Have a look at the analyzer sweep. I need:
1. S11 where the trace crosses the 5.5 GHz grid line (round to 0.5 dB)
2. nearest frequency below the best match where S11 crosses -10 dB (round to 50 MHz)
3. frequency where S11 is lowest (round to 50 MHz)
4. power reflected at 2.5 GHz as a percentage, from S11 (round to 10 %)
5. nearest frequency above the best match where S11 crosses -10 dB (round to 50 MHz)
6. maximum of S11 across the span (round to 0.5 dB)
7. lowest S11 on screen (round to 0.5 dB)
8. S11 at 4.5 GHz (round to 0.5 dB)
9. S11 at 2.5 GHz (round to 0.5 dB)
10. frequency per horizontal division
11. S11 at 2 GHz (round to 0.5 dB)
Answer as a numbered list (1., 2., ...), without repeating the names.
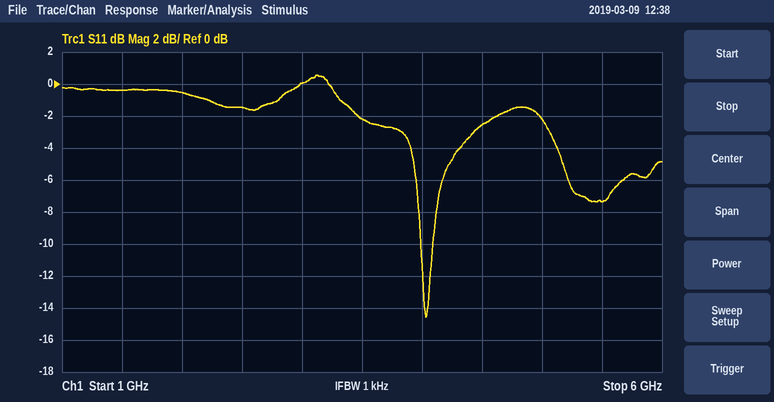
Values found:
1. -7.5 dB
2. 4.00 GHz
3. 4.05 GHz
4. 70 %
5. 4.10 GHz
6. 0.5 dB
7. -14.5 dB
8. -2.5 dB
9. -1.5 dB
10. 500 MHz
11. -0.5 dB
